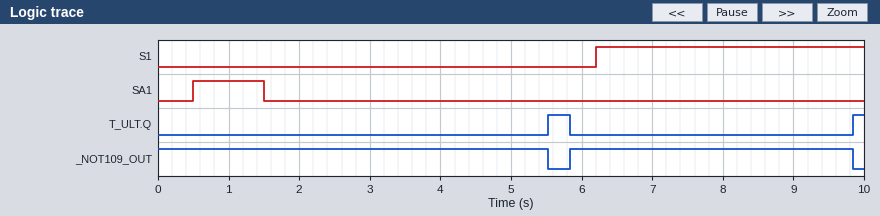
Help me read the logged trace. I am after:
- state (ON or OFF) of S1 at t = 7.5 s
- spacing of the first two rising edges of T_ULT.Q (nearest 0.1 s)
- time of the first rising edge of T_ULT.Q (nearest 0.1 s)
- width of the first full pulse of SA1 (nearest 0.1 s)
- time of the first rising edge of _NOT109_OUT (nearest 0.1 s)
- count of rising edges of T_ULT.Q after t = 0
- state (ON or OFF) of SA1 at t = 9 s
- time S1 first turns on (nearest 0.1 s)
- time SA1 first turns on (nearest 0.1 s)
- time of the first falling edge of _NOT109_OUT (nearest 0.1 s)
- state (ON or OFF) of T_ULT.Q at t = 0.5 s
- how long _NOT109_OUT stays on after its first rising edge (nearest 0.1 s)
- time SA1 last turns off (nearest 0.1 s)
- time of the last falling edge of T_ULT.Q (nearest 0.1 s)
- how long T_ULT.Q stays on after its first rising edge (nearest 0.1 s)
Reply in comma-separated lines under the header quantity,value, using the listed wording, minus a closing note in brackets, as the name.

quantity,value
state (ON or OFF) of S1 at t = 7.5 s,ON
spacing of the first two rising edges of T_ULT.Q,4.3 s
time of the first rising edge of T_ULT.Q,5.5 s
width of the first full pulse of SA1,1.0 s
time of the first rising edge of _NOT109_OUT,5.8 s
count of rising edges of T_ULT.Q after t = 0,2
state (ON or OFF) of SA1 at t = 9 s,OFF
time S1 first turns on,6.2 s
time SA1 first turns on,0.5 s
time of the first falling edge of _NOT109_OUT,5.5 s
state (ON or OFF) of T_ULT.Q at t = 0.5 s,OFF
how long _NOT109_OUT stays on after its first rising edge,4.0 s
time SA1 last turns off,1.5 s
time of the last falling edge of T_ULT.Q,5.8 s
how long T_ULT.Q stays on after its first rising edge,0.3 s
